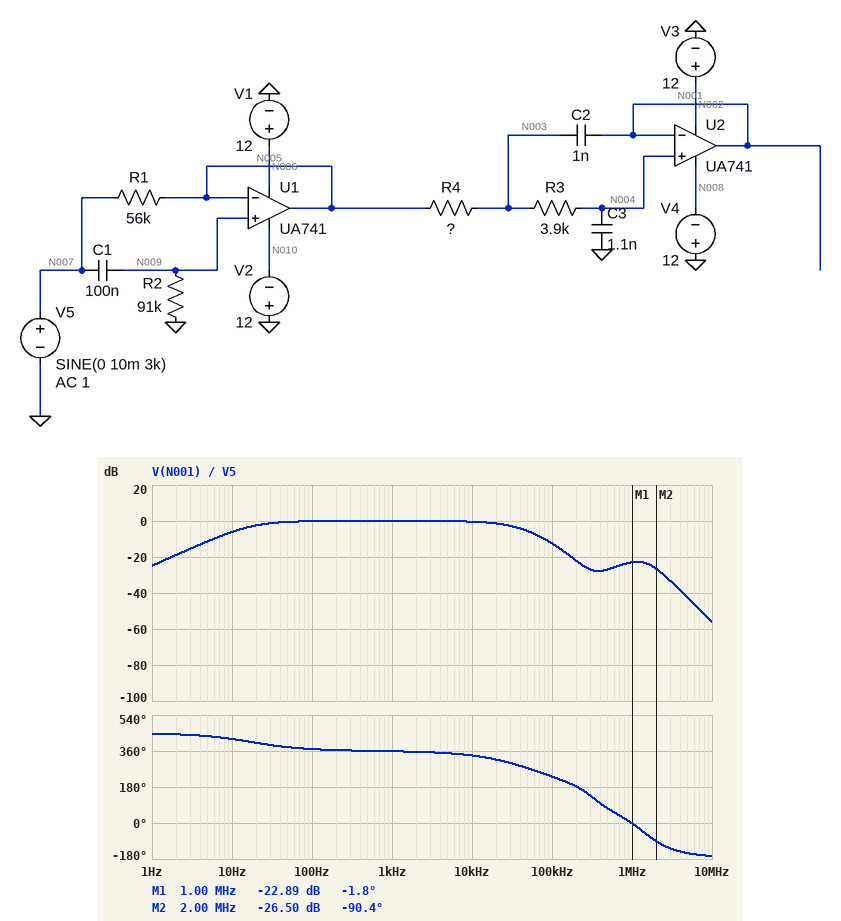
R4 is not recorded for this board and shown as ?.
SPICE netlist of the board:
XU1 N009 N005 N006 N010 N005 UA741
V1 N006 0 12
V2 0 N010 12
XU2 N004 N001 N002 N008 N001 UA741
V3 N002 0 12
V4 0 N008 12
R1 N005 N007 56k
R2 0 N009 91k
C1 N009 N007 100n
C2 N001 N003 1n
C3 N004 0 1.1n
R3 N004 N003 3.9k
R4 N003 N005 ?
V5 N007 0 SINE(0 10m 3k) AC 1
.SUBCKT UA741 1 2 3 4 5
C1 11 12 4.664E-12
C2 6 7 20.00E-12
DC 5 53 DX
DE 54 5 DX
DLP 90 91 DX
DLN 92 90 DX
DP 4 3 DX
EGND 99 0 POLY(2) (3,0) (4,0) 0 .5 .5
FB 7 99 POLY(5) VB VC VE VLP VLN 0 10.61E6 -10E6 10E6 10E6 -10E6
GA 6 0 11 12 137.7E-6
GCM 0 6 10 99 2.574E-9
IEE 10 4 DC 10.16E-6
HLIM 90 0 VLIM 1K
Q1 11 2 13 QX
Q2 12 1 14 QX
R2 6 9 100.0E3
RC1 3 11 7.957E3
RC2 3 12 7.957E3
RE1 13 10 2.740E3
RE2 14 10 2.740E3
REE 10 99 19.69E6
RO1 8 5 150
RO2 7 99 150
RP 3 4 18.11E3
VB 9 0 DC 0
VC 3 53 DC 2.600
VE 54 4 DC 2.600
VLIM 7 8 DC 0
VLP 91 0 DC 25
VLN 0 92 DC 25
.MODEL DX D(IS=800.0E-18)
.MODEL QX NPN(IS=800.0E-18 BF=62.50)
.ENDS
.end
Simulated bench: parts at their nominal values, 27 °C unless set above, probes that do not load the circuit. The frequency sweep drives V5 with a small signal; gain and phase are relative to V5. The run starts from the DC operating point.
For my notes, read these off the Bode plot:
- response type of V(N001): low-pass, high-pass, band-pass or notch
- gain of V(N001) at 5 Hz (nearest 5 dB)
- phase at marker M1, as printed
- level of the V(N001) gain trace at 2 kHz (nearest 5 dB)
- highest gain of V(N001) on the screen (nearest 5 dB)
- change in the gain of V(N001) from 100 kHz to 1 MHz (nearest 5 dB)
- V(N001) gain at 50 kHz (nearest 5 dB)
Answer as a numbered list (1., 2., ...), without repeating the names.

1. band-pass
2. -10 dB
3. -1.8 deg
4. 0 dB
5. 0 dB
6. -10 dB
7. -5 dB
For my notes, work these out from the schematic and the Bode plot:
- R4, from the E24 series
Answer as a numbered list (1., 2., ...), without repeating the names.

1. 1.6 kΩ
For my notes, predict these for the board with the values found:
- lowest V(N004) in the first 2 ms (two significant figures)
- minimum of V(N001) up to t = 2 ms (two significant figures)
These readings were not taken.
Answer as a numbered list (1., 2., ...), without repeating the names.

1. -18 mV
2. -18 mV
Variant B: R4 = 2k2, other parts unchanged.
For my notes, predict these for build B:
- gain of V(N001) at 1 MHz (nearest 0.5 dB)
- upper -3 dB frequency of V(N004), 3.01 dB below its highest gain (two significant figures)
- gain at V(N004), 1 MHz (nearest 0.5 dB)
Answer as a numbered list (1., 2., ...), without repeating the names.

1. -25.5 dB
2. 30 kHz
3. -58.5 dB
